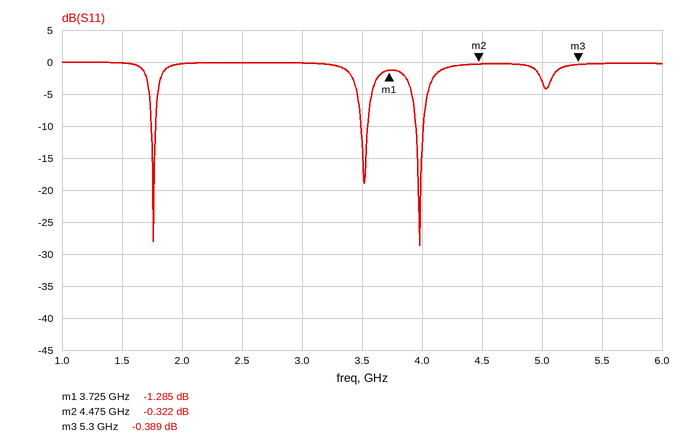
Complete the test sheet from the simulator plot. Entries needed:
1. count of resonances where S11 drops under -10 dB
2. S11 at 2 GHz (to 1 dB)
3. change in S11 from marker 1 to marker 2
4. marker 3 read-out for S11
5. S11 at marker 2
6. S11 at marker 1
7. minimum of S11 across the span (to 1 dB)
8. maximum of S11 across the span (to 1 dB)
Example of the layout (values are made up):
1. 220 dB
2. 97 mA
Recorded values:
1. 3
2. 0 dB
3. 0.963 dB
4. -0.389 dB
5. -0.322 dB
6. -1.285 dB
7. -29 dB
8. 0 dB
